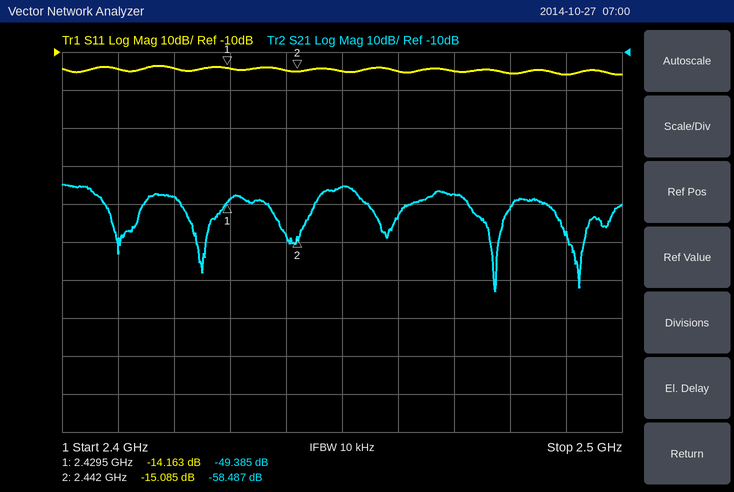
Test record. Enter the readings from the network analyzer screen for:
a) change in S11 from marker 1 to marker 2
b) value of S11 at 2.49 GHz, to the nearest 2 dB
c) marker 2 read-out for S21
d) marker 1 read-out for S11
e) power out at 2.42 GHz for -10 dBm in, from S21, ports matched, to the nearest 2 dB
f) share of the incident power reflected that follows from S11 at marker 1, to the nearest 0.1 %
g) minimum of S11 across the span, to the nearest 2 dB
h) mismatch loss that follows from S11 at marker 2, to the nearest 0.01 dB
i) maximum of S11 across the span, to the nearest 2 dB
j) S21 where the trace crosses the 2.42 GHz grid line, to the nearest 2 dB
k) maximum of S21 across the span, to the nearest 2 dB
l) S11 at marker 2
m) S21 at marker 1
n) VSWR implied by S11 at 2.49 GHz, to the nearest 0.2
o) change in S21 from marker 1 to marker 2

-0.922 dB
-16 dB
-58.487 dB
-14.163 dB
-58 dBm
3.8 %
-16 dB
0.14 dB
-14 dB
-48 dB
-44 dB
-15.085 dB
-49.385 dB
1.4
-9.102 dB
